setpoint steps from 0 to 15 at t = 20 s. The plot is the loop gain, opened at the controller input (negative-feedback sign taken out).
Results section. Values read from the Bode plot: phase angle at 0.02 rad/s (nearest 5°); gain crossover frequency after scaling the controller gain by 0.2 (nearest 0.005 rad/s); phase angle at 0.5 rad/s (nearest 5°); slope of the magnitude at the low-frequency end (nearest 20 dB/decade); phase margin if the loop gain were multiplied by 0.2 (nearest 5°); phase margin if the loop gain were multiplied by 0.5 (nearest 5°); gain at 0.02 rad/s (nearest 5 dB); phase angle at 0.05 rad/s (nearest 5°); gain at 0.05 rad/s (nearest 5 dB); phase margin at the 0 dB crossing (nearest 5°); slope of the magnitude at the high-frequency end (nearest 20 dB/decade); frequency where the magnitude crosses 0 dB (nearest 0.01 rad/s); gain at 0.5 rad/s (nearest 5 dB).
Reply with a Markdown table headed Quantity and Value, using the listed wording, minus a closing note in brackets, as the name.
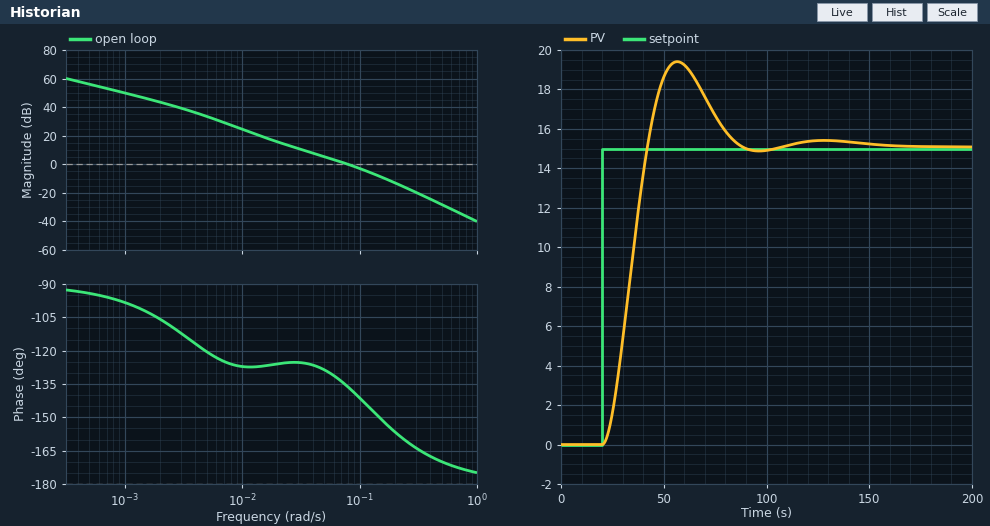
| Quantity | Value |
|---|---|
| phase angle at 0.02 rad/s | -125° |
| gain crossover frequency after scaling the controller gain by 0.2 | 0.025 rad/s |
| phase angle at 0.5 rad/s | -170° |
| slope of the magnitude at the low-frequency end | -20 dB/decade |
| phase margin if the loop gain were multiplied by 0.2 | 55° |
| phase margin if the loop gain were multiplied by 0.5 | 50° |
| gain at 0.02 rad/s | 15 dB |
| phase angle at 0.05 rad/s | -130° |
| gain at 0.05 rad/s | 5 dB |
| phase margin at the 0 dB crossing | 45° |
| slope of the magnitude at the high-frequency end | -40 dB/decade |
| frequency where the magnitude crosses 0 dB | 0.08 rad/s |
| gain at 0.5 rad/s | -30 dB |
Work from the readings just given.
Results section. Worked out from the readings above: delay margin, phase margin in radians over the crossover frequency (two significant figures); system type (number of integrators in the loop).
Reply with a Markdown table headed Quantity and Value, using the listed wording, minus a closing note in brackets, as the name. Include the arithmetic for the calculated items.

| Quantity | Value |
|---|---|
| delay margin, phase margin in radians over the crossover frequency | 45 × π / 180 / 0.08 = 9.8 s |
| system type | 1 |
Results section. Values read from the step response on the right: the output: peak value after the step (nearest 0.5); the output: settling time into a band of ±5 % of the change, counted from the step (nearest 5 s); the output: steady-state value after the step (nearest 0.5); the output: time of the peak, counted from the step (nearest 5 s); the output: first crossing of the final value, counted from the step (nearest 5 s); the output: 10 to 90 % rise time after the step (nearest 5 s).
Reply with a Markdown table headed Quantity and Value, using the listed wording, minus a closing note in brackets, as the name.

| Quantity | Value |
|---|---|
| the output: peak value after the step | 19.5 |
| the output: settling time into a band of ±5 % of the change, counted from the step | 60 s |
| the output: steady-state value after the step | 15.0 |
| the output: time of the peak, counted from the step | 35 s |
| the output: first crossing of the final value, counted from the step | 20 s |
| the output: 10 to 90 % rise time after the step | 15 s |
